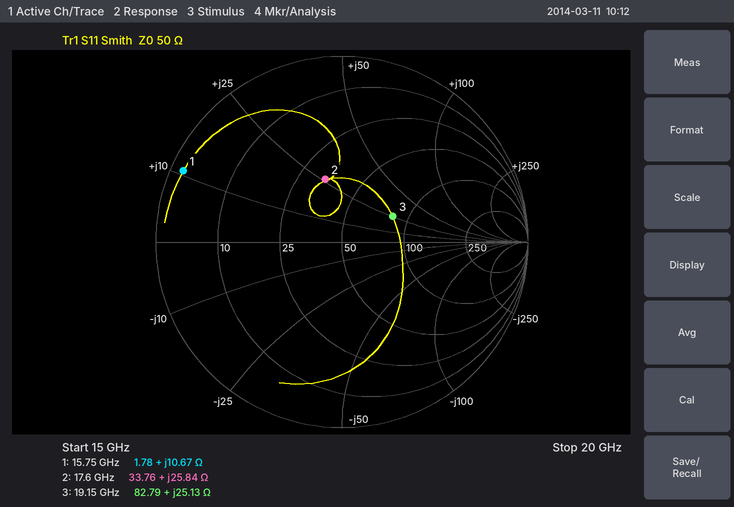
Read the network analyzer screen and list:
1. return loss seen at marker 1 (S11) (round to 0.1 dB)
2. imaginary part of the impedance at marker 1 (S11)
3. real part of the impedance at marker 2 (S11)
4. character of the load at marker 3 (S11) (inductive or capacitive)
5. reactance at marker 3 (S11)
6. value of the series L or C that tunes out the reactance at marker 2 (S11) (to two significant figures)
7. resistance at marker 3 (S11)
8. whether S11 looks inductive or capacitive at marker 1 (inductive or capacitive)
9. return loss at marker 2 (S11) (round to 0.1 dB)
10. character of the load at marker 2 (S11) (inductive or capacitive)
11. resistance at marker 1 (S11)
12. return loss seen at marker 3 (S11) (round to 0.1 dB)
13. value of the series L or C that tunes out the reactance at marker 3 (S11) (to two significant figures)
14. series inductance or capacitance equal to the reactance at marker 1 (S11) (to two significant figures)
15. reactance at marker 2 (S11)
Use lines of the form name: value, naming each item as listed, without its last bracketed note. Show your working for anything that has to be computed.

return loss seen at marker 1 (S11): 0.6 dB
imaginary part of the impedance at marker 1: +10.67 Ω
real part of the impedance at marker 2: 33.76 Ω
character of the load at marker 3 (S11): inductive
reactance at marker 3: +25.13 Ω
value of the series L or C that tunes out the reactance at marker 2 (S11): C = 1/(2π × 17.6 GHz × 25.84 Ω) ≈ 350 fF
resistance at marker 3: 82.79 Ω
whether S11 looks inductive or capacitive at marker 1: inductive
return loss at marker 2 (S11): 9.2 dB
character of the load at marker 2 (S11): inductive
resistance at marker 1: 1.78 Ω
return loss seen at marker 3 (S11): 10.3 dB
value of the series L or C that tunes out the reactance at marker 3 (S11): C = 1/(2π × 19.15 GHz × 25.13 Ω) ≈ 331 fF, so 330 fF to two significant figures
series inductance or capacitance equal to the reactance at marker 1 (S11): L = 10.67 Ω/(2π × 15.75 GHz) ≈ 108 pH, so 110 pH to two significant figures
reactance at marker 2: +25.84 Ω
